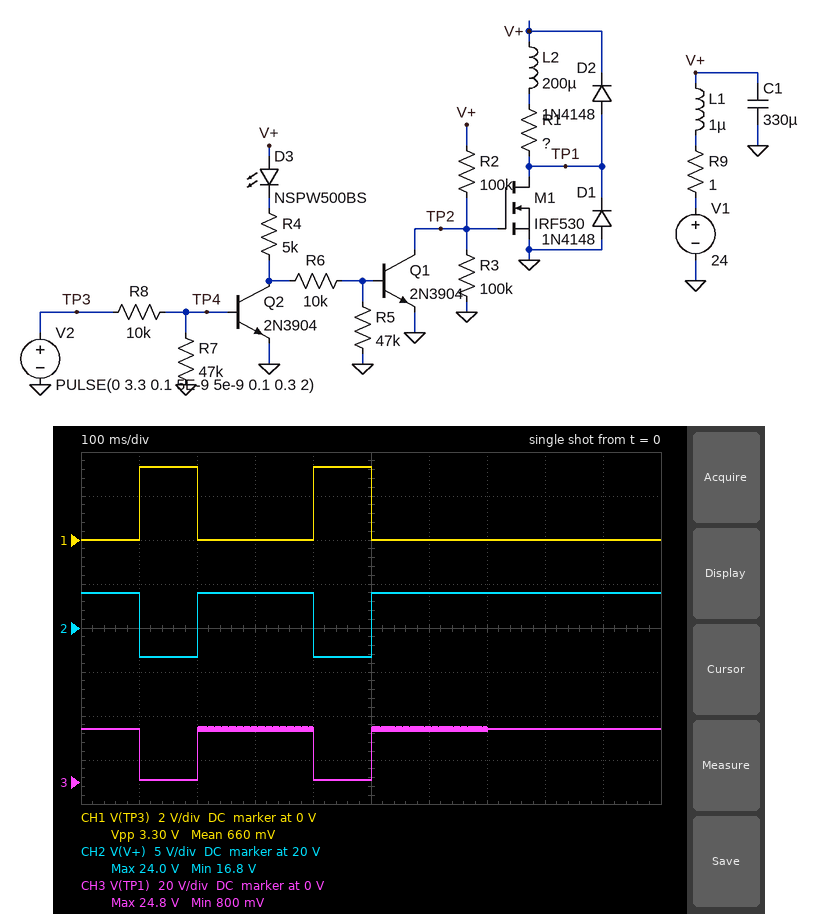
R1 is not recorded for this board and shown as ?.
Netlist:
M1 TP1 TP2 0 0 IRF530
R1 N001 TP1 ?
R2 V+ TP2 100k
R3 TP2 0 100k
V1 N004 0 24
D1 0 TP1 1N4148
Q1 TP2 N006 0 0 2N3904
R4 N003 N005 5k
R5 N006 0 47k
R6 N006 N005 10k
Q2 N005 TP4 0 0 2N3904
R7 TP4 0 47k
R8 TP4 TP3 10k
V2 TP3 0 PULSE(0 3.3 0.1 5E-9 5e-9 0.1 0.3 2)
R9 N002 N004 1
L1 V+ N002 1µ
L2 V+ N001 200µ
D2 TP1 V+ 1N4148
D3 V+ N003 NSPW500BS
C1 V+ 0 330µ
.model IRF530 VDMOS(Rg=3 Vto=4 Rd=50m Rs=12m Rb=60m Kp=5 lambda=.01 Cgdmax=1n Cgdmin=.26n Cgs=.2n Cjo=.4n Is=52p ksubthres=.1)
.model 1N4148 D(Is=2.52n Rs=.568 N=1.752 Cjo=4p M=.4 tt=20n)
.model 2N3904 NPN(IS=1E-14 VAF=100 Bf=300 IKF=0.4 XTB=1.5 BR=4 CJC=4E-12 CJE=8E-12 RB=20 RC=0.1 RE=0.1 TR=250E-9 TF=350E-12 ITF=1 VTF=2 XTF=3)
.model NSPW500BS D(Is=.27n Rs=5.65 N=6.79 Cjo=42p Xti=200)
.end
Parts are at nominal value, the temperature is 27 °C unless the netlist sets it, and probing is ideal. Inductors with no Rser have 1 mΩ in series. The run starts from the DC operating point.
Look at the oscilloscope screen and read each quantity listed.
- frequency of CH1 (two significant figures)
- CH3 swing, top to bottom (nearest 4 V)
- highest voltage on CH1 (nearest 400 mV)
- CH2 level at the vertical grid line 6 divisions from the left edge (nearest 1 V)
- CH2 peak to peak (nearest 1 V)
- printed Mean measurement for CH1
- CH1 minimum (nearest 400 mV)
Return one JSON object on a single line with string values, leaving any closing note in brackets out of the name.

{"frequency of CH1": "3.3 Hz", "CH3 swing, top to bottom": "24 V", "highest voltage on CH1": "3.2 V", "CH2 level at the vertical grid line 6 divisions from the left edge": "24 V", "CH2 peak to peak": "7 V", "printed Mean measurement for CH1": "660 mV", "CH1 minimum": "0 V"}
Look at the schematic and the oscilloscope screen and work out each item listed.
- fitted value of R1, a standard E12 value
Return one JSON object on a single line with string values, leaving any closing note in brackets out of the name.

{"fitted value of R1, a standard E12 value": "2.2 Ω"}
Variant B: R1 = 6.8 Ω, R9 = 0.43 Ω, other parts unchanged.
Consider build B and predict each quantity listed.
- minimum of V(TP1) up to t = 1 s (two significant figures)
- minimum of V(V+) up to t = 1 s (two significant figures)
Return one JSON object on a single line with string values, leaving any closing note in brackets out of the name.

{"minimum of V(TP1) up to t = 1 s": "290 mV", "minimum of V(V+) up to t = 1 s": "23 V"}
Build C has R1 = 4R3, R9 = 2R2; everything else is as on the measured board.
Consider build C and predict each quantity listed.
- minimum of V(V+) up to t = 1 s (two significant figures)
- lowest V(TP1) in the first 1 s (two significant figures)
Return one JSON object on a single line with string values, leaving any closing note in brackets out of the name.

{"minimum of V(V+) up to t = 1 s": "16 V", "lowest V(TP1) in the first 1 s": "410 mV"}
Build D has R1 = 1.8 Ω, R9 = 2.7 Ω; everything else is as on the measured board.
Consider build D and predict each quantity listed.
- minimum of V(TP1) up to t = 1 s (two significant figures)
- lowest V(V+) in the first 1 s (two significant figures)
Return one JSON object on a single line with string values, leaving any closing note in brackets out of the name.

{"minimum of V(TP1) up to t = 1 s": "770 mV", "lowest V(V+) in the first 1 s": "11 V"}
